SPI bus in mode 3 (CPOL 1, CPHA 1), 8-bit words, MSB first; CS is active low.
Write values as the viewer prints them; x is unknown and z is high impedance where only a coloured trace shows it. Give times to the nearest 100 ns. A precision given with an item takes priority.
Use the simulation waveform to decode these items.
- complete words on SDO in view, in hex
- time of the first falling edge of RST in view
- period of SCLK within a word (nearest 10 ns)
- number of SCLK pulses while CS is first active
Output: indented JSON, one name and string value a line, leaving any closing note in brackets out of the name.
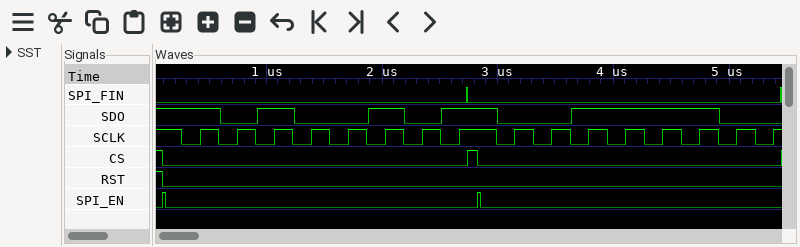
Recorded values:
{
  "complete words on SDO in view, in hex": "A5, 3C",
  "time of the first falling edge of RST in view": "100 ns",
  "period of SCLK within a word": "320 ns",
  "number of SCLK pulses while CS is first active": "8"
}
